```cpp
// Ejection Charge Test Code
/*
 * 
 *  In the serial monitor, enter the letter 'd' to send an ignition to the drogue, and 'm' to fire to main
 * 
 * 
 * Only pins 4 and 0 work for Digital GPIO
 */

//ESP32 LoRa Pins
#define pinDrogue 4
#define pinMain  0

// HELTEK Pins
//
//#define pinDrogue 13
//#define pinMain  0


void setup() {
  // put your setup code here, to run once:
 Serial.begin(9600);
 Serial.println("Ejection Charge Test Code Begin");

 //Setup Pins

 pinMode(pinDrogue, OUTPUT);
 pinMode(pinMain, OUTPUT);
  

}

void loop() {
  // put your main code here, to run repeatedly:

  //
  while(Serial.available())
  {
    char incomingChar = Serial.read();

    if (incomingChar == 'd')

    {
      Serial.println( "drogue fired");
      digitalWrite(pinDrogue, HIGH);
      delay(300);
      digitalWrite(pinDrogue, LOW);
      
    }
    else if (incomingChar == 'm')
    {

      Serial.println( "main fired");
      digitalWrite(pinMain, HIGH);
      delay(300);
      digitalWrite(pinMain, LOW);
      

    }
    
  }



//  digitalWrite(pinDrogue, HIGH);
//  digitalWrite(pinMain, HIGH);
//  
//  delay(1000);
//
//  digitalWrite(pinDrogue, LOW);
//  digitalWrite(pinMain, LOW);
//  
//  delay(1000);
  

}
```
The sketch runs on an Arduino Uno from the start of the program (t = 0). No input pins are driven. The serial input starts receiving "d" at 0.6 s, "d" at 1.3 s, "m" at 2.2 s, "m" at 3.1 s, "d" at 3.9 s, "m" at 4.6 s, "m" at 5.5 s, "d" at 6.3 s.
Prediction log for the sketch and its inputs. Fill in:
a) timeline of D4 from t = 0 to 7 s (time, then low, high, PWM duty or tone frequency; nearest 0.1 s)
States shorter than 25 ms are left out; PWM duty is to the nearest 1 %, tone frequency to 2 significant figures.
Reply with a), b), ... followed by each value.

a) 0 s low; 0.6 s high; 0.9 s low; 1.3 s high; 1.6 s low; 3.9 s high; 4.2 s low; 6.3 s high; 6.6 s low
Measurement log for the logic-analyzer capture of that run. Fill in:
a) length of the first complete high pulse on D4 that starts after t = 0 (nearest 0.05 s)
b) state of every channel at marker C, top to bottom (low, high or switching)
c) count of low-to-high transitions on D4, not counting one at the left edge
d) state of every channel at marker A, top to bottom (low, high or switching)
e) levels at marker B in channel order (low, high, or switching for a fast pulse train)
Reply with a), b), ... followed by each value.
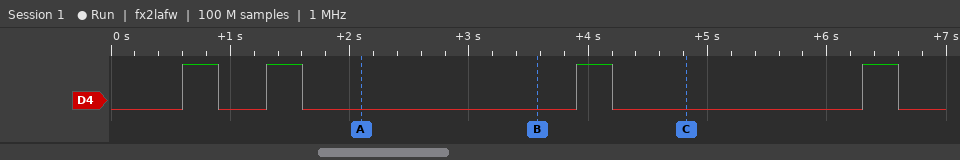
a) 0.30 s
b) D4 low
c) 4
d) D4 low
e) D4 low
